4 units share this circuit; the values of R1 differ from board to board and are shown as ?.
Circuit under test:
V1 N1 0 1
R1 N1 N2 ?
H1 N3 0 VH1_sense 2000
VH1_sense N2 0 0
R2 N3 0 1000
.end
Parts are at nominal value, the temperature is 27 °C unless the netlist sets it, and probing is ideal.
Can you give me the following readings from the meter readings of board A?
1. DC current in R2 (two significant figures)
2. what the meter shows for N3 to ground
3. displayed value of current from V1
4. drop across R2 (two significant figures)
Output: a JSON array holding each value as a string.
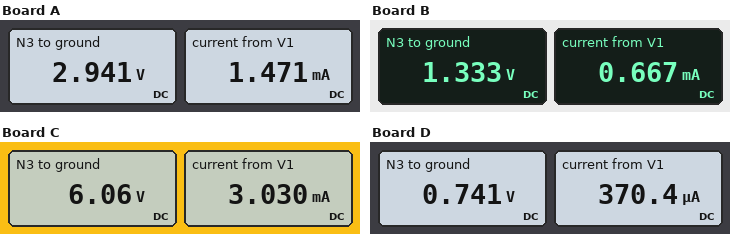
["2.9 mA", "2.941 V", "1.471 mA", "2.9 V"]
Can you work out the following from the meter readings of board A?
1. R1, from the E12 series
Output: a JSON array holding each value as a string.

["680 Ω"]
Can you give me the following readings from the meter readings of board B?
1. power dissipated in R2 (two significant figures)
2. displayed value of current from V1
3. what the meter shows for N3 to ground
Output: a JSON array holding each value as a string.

["1.8 mW", "0.667 mA", "1.333 V"]
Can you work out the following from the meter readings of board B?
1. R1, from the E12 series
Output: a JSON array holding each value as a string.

["1.5 kΩ"]
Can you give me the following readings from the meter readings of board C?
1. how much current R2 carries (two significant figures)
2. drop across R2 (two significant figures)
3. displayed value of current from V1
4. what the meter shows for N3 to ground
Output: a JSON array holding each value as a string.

["6.1 mA", "6.1 V", "3.030 mA", "6.06 V"]
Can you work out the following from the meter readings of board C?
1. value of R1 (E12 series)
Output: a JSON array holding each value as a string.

["330 Ω"]
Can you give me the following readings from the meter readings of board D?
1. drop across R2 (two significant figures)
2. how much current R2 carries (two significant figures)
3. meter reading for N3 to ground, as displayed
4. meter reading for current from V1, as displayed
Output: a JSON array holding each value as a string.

["740 mV", "740 µA", "0.741 V", "370.4 µA"]
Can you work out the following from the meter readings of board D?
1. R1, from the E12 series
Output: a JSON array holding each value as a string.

["2.7 kΩ"]
